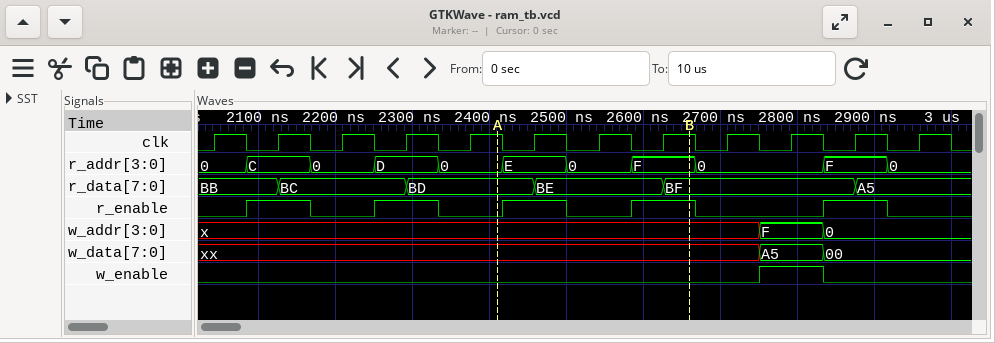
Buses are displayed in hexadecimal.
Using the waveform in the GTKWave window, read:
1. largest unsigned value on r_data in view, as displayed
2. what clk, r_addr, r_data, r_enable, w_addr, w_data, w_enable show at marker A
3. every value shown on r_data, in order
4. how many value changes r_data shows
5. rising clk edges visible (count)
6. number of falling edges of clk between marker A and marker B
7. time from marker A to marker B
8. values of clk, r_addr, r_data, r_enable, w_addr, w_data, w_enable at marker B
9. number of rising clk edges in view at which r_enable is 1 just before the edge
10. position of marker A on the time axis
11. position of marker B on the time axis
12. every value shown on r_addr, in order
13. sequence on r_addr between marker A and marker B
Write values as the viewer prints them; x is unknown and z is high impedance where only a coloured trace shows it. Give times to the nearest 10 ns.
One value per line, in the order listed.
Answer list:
BF
clk=1, r_addr=0, r_data=BD, r_enable=0, w_addr=x, w_data=xx, w_enable=0
BB, BC, BD, BE, BF, A5
5
12
3
250 ns
clk=1, r_addr=F, r_data=BF, r_enable=1, w_addr=x, w_data=xx, w_enable=0
5
2410 ns
2660 ns
0, C, 0, D, 0, E, 0, F, 0, F, 0
0, E, 0, F
